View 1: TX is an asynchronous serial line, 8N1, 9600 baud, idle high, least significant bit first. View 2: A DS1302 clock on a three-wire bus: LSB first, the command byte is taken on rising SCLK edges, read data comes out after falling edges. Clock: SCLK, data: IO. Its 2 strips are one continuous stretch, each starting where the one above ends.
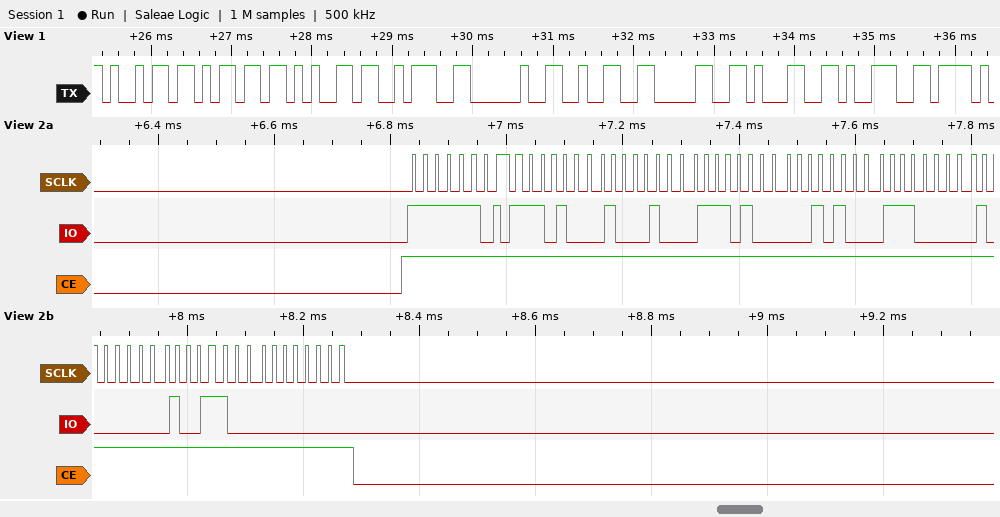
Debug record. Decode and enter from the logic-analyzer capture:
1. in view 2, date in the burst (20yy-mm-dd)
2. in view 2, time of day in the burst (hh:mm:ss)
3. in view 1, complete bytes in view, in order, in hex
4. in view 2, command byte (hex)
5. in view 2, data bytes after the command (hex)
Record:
2019-07-14
17:11:17
69 6D 65 3A 20 32 30 31 39
0xBF
17 11 17 14 07 01 19 00
